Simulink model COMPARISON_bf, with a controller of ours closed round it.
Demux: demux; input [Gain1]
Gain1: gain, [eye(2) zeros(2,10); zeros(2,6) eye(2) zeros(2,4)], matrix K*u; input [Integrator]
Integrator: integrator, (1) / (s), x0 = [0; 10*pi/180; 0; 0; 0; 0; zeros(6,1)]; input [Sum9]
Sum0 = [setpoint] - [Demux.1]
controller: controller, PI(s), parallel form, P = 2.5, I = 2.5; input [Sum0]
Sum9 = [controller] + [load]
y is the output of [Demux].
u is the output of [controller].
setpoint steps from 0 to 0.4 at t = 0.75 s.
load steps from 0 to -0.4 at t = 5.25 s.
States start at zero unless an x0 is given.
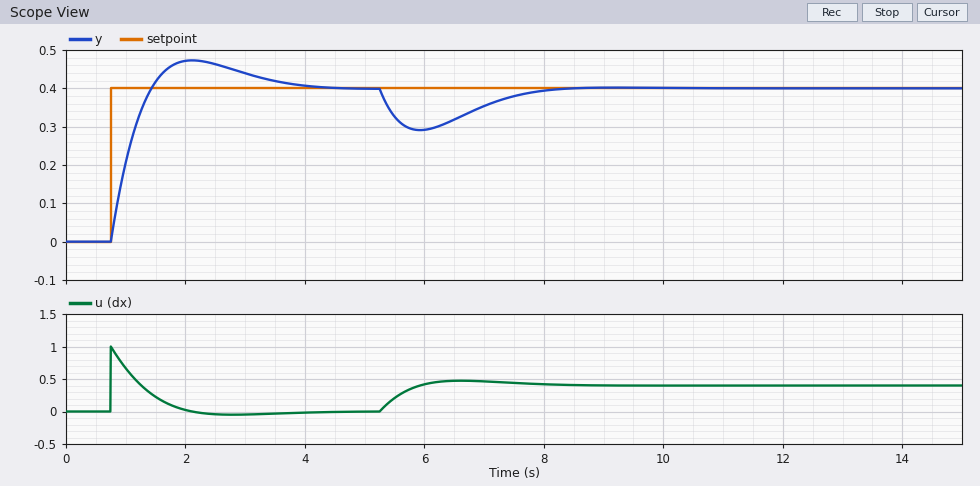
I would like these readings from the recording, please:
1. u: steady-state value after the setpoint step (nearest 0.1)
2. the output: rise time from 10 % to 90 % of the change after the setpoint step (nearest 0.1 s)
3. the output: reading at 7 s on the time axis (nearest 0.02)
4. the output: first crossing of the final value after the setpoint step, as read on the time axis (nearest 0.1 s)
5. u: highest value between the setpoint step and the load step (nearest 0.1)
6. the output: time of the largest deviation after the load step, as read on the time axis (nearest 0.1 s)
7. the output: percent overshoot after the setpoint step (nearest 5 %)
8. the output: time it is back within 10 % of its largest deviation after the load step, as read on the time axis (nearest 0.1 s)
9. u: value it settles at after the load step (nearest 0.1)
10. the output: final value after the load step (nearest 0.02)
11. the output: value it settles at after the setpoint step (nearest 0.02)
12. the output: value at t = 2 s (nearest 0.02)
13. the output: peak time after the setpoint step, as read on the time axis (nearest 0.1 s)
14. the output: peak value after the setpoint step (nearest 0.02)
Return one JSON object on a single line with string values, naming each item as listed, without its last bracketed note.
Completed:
{"u: steady-state value after the setpoint step": "0.0", "the output: rise time from 10 % to 90 % of the change after the setpoint step": "0.5 s", "the output: reading at 7 s on the time axis": "0.36", "the output: first crossing of the final value after the setpoint step, as read on the time axis": "1.4 s", "u: highest value between the setpoint step and the load step": "1.0", "the output: time of the largest deviation after the load step, as read on the time axis": "5.9 s", "the output: percent overshoot after the setpoint step": "20 %", "the output: time it is back within 10 % of its largest deviation after the load step, as read on the time axis": "7.8 s", "u: value it settles at after the load step": "0.4", "the output: final value after the load step": "0.40", "the output: value it settles at after the setpoint step": "0.40", "the output: value at t = 2 s": "0.48", "the output: peak time after the setpoint step, as read on the time axis": "2.1 s", "the output: peak value after the setpoint step": "0.48"}
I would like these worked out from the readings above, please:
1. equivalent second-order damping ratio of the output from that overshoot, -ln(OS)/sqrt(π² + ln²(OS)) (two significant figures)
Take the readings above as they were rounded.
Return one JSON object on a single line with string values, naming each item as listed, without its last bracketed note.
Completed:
{"equivalent second-order damping ratio of the output from that overshoot, -ln(OS)/sqrt(π² + ln²(OS))": "0.46"}
